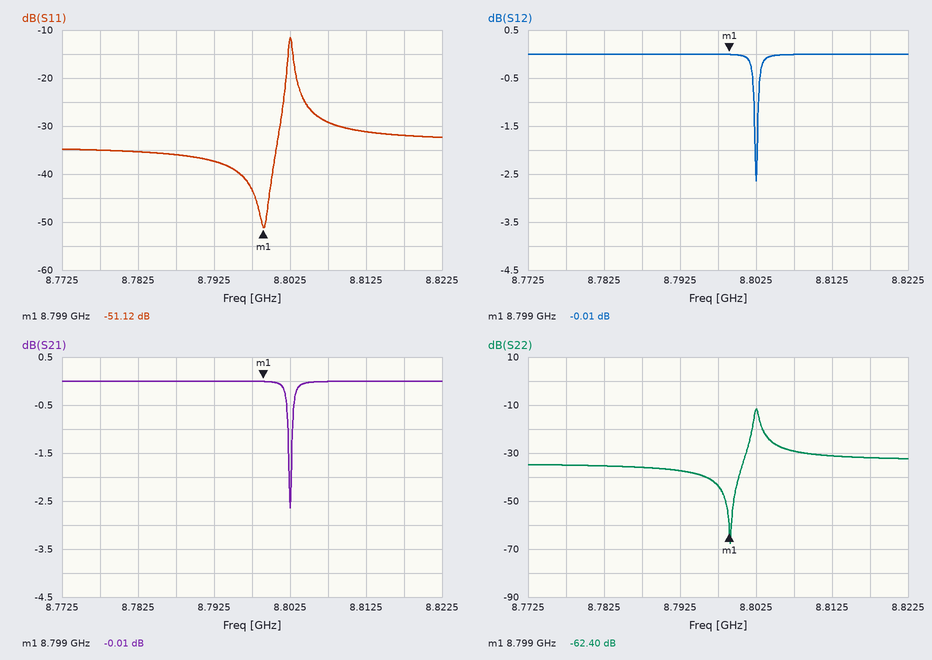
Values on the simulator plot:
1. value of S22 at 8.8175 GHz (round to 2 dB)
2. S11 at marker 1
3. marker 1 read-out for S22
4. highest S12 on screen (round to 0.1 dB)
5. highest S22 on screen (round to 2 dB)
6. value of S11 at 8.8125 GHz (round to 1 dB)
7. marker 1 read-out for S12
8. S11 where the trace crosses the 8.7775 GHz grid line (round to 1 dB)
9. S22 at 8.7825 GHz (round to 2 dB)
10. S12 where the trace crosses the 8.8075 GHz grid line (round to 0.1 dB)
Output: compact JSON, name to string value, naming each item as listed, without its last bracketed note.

{"value of S22 at 8.8175 GHz": "-32 dB", "S11 at marker 1": "-51.12 dB", "marker 1 read-out for S22": "-62.40 dB", "highest S12 on screen": "0.0 dB", "highest S22 on screen": "-12 dB", "value of S11 at 8.8125 GHz": "-31 dB", "marker 1 read-out for S12": "-0.01 dB", "S11 where the trace crosses the 8.7775 GHz grid line": "-35 dB", "S22 at 8.7825 GHz": "-36 dB", "S12 where the trace crosses the 8.8075 GHz grid line": "0.0 dB"}
